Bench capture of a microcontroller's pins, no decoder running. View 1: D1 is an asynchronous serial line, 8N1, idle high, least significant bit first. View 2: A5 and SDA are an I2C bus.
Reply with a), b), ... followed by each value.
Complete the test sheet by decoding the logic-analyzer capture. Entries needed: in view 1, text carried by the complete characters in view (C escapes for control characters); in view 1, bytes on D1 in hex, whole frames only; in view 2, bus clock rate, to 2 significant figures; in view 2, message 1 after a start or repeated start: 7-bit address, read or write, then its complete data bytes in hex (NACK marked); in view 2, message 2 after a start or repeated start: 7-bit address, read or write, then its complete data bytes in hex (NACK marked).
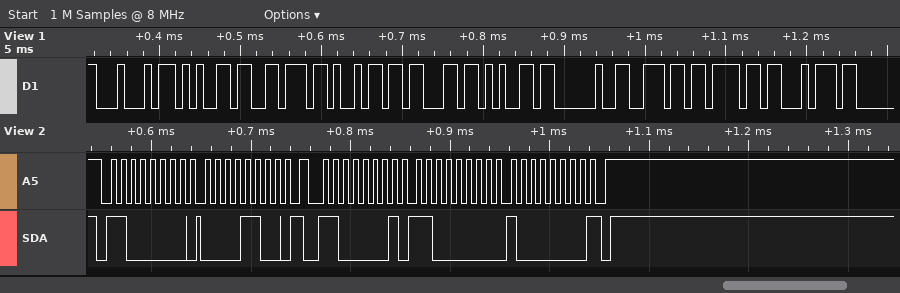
a) "Device not"
b) 44 65 76 69 63 65 20 6E 6F 74
c) 100 kHz
d) 0x60 write: 0C
e) 0x60 read: C0 80 NACK
